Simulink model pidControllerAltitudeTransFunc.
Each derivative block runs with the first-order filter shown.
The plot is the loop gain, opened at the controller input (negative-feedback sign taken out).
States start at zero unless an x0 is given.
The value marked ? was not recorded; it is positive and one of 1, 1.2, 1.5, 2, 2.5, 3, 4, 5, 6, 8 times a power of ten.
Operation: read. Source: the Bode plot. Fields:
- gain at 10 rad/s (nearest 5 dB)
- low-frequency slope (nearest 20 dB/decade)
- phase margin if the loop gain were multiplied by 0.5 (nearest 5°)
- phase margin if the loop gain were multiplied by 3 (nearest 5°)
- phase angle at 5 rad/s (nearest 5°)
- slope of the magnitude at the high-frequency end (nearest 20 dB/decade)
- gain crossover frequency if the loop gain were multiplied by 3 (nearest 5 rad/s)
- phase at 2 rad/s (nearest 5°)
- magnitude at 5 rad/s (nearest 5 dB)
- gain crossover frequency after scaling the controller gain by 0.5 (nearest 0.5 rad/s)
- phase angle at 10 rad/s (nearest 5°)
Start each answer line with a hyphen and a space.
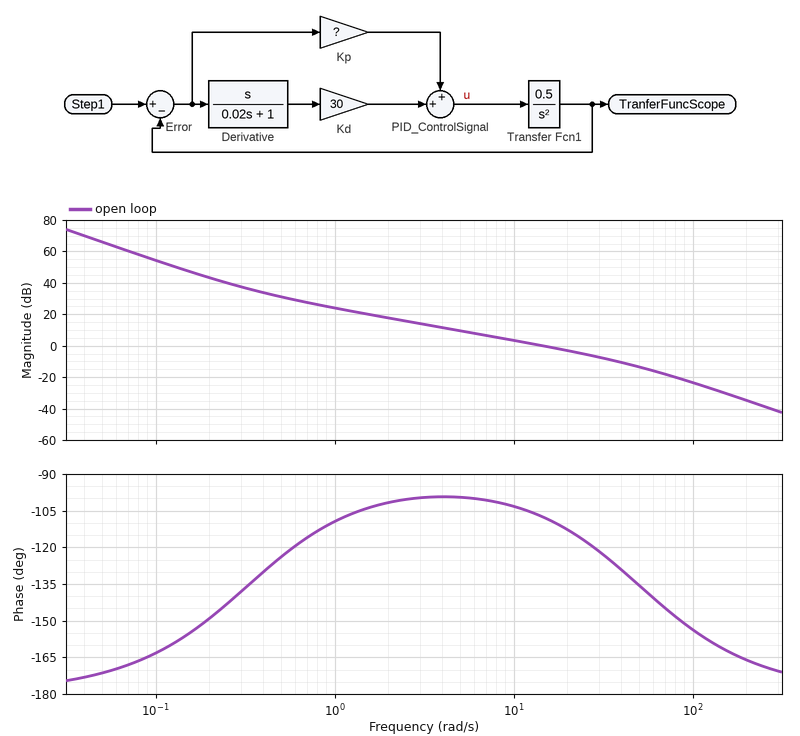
- 5 dB
- -40 dB/decade
- 80°
- 55°
- -100°
- -40 dB/decade
- 35 rad/s
- -100°
- 10 dB
- 7.5 rad/s
- -105°
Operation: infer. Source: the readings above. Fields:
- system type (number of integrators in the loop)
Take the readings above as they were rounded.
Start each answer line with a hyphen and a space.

- 2
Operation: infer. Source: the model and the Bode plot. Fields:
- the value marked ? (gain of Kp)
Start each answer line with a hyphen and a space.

- 10
